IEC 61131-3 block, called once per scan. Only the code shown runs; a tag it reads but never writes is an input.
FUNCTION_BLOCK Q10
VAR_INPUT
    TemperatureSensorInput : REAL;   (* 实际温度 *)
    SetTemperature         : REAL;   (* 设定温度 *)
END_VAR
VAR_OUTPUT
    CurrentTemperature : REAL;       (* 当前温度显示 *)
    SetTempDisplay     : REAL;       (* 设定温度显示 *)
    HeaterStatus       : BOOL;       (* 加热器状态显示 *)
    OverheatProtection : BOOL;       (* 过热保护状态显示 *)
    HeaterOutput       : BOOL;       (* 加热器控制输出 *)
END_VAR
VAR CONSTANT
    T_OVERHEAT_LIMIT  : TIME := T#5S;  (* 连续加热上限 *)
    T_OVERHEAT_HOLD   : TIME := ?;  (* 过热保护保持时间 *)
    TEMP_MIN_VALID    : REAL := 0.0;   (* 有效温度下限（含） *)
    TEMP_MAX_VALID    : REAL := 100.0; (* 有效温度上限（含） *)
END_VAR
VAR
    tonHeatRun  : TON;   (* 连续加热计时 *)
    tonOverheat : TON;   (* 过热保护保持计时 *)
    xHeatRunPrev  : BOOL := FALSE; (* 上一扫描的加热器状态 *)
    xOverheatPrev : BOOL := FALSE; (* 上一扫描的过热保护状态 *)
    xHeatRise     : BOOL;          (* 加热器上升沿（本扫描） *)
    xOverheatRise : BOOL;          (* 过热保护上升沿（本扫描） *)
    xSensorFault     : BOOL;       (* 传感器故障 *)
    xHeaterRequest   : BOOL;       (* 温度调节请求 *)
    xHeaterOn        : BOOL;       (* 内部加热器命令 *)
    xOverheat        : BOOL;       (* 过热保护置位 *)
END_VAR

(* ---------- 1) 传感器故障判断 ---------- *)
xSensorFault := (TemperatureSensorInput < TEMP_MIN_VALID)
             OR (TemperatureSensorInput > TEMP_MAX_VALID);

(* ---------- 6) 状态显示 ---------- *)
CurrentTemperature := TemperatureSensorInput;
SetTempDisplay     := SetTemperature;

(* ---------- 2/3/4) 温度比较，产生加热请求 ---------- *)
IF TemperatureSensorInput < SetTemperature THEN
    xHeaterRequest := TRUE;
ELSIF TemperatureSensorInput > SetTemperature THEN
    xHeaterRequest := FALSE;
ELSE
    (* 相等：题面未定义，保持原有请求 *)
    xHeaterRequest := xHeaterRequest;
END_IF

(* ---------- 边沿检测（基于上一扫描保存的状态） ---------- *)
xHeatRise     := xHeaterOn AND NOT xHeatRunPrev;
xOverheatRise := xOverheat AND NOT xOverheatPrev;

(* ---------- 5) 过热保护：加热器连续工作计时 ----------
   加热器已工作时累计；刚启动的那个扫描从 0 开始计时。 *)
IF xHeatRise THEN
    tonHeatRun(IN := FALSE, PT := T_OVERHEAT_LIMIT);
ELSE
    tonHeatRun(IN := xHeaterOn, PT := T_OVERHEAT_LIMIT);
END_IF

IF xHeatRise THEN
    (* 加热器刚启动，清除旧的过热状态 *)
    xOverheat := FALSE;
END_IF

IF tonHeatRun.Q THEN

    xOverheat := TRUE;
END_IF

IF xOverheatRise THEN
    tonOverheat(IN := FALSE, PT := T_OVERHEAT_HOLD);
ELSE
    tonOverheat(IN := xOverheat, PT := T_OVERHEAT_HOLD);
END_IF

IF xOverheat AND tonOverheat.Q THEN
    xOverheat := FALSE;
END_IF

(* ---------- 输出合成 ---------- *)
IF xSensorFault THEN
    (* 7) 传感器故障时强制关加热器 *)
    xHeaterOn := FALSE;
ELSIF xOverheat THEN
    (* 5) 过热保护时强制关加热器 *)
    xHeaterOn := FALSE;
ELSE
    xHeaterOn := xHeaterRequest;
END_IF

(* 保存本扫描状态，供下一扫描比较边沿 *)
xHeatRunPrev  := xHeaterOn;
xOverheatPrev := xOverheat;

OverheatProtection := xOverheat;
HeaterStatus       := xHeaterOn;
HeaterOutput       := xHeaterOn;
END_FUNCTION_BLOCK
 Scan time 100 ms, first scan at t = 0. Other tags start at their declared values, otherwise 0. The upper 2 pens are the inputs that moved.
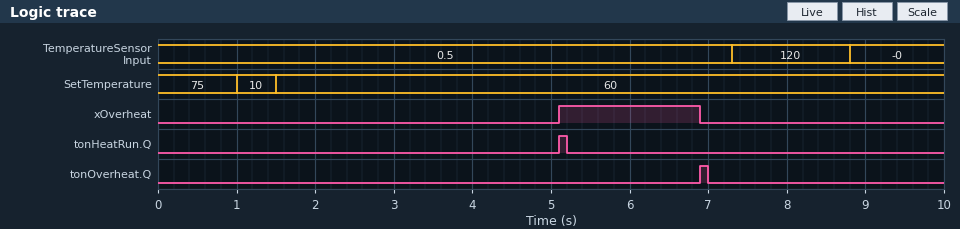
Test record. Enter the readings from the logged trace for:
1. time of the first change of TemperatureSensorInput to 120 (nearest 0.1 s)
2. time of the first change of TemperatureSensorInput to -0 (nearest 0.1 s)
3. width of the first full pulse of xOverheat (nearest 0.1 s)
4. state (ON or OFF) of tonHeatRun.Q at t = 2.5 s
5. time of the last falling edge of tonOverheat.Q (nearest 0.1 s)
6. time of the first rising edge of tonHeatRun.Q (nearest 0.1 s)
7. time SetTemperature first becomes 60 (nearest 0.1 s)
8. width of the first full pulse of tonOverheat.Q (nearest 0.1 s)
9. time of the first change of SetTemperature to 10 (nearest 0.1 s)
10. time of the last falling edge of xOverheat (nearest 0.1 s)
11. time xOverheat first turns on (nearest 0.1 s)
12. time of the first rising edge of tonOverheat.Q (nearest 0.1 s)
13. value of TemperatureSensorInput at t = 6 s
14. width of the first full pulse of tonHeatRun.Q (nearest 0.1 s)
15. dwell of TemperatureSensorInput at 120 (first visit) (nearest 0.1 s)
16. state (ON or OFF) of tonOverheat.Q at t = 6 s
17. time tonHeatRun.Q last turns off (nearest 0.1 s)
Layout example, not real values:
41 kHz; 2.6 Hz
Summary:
7.3 s; 8.8 s; 1.8 s; OFF; 7.0 s; 5.1 s; 1.5 s; 0.1 s; 1.0 s; 6.9 s; 5.1 s; 6.9 s; 0.5; 0.1 s; 1.5 s; OFF; 5.2 s
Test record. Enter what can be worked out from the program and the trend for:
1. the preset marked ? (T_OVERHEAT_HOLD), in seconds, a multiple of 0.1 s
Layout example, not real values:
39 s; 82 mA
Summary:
1.8 s
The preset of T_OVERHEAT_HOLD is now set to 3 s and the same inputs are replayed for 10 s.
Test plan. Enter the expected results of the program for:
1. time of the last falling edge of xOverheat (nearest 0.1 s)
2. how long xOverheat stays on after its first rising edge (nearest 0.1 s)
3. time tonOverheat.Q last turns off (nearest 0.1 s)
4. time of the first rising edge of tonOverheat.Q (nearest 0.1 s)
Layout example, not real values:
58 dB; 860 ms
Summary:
8.1 s; 3.0 s; 8.2 s; 8.1 s
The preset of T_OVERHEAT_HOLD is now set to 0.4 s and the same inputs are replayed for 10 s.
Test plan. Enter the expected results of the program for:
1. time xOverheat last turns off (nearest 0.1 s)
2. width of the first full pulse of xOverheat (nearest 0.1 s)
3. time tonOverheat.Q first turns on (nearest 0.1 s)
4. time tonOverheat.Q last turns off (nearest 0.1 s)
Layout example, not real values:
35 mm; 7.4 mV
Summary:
5.5 s; 0.4 s; 5.5 s; 5.6 s
